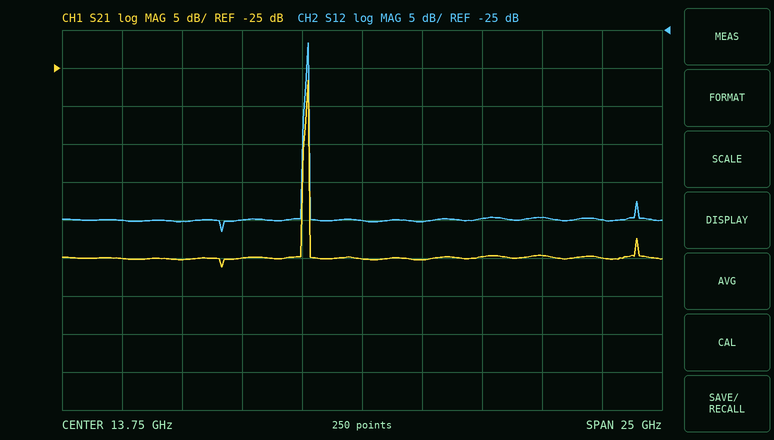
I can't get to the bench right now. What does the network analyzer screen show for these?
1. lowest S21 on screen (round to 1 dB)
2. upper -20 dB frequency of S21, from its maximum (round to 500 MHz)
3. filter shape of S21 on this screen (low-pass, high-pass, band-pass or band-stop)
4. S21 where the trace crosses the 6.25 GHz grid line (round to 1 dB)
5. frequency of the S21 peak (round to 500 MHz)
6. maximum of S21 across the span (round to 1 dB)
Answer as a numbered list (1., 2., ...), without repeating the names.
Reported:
1. -51 dB
2. 11.5 GHz
3. band-pass
4. -50 dB
5. 11.5 GHz
6. -27 dB
